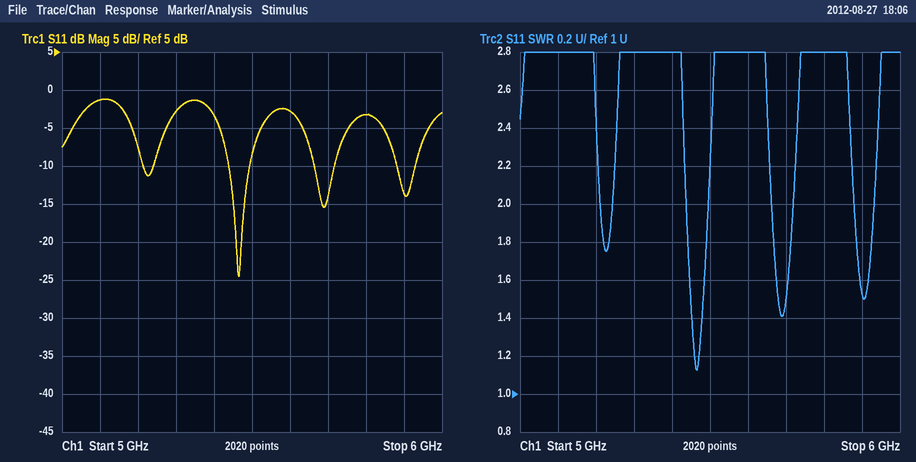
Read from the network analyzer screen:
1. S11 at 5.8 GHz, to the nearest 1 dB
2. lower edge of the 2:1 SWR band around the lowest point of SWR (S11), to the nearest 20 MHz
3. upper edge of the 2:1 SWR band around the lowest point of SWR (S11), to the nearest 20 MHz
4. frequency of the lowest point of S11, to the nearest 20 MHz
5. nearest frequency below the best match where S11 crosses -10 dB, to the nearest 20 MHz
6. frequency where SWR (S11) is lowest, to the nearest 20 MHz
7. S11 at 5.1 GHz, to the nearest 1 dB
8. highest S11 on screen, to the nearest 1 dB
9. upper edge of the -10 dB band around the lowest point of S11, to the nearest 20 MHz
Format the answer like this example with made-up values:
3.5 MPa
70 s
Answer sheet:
-3 dB
5.44 GHz
5.50 GHz
5.46 GHz
5.44 GHz
5.46 GHz
-1 dB
-1 dB
5.50 GHz
